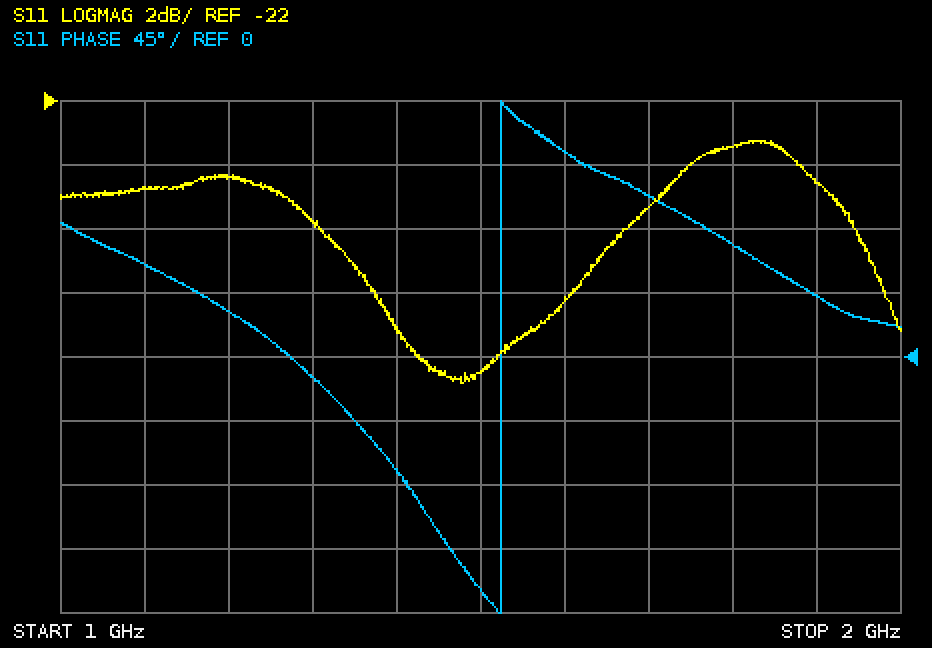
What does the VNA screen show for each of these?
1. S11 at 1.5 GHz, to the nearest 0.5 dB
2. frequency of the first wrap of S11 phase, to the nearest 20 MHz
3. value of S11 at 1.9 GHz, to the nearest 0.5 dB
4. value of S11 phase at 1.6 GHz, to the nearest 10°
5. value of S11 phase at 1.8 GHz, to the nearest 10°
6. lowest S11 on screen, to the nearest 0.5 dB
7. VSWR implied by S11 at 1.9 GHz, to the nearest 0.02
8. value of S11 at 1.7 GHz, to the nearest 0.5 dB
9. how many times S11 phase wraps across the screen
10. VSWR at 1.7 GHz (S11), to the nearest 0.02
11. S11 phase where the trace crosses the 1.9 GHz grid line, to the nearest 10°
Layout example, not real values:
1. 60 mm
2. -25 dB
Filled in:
1. -30.5 dB
2. 1.52 GHz
3. -24.5 dB
4. 140°
5. 80°
6. -31.0 dB
7. 1.12
8. -25.5 dB
9. 1
10. 1.12
11. 40°
